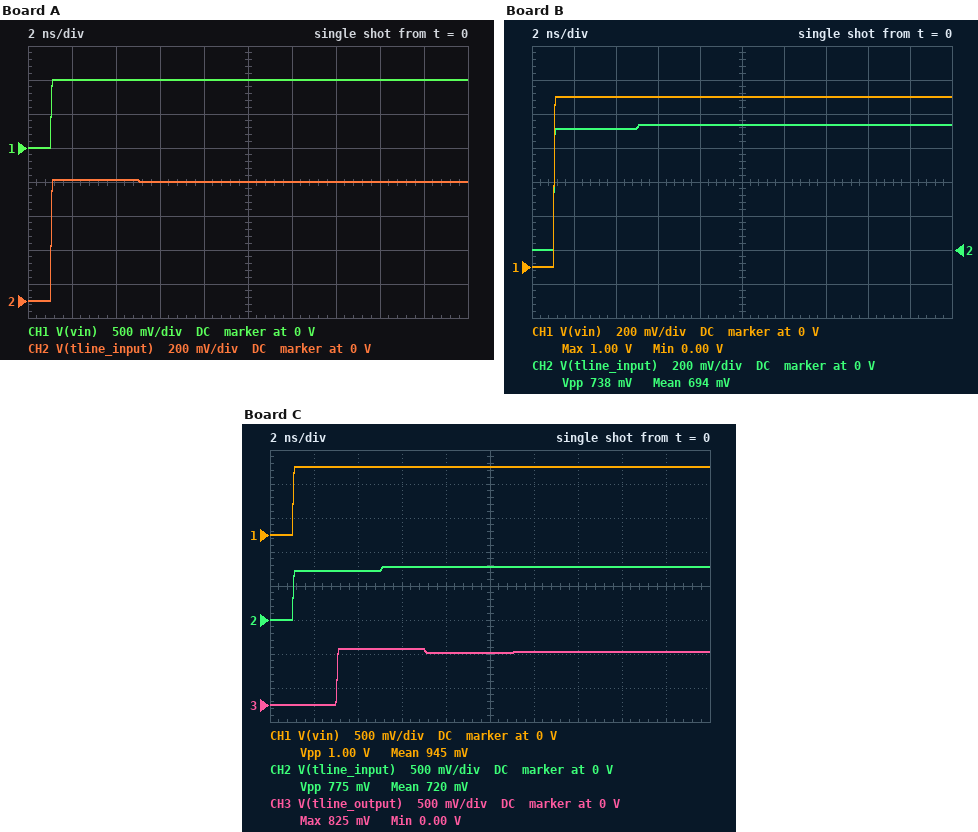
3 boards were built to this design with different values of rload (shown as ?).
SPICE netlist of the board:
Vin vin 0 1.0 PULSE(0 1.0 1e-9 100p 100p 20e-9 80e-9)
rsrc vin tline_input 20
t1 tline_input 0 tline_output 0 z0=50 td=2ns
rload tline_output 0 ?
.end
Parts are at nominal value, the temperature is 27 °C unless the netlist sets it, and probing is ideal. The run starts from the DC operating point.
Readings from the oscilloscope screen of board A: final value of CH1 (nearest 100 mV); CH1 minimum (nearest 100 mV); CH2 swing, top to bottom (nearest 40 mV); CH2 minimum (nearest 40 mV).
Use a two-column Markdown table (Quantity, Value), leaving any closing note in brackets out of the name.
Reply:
| Quantity | Value |
|---|---|
| final value of CH1 | 1.0 V |
| CH1 minimum | 0 V |
| CH2 swing, top to bottom | 720 mV |
| CH2 minimum | 0 V |
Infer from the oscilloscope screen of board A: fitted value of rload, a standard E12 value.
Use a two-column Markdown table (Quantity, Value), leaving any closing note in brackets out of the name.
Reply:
| Quantity | Value |
|---|---|
| fitted value of rload, a standard E12 value | 47 Ω |
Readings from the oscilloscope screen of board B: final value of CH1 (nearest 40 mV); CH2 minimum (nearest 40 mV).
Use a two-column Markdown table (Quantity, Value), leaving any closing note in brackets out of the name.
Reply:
| Quantity | Value |
|---|---|
| final value of CH1 | 1.00 V |
| CH2 minimum | 0 V |
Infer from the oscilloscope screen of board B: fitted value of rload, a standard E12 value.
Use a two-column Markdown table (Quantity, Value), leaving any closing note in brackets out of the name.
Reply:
| Quantity | Value |
|---|---|
| fitted value of rload, a standard E12 value | 56 Ω |
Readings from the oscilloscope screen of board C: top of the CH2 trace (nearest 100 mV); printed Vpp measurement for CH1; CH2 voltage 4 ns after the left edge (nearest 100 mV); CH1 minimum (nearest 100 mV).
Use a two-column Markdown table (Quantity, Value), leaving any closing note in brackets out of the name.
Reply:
| Quantity | Value |
|---|---|
| top of the CH2 trace | 800 mV |
| printed Vpp measurement for CH1 | 1.00 V |
| CH2 voltage 4 ns after the left edge | 700 mV |
| CH1 minimum | 0 V |
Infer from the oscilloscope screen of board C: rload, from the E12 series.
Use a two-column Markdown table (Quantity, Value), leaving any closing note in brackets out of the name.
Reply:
| Quantity | Value |
|---|---|
| rload, from the E12 series | 68 Ω |
